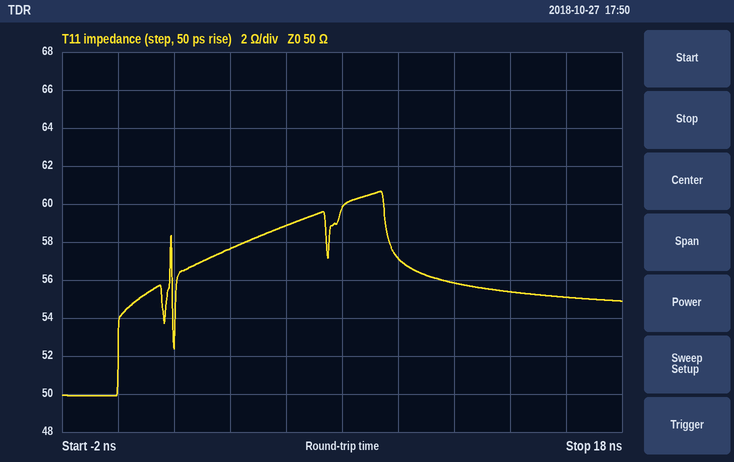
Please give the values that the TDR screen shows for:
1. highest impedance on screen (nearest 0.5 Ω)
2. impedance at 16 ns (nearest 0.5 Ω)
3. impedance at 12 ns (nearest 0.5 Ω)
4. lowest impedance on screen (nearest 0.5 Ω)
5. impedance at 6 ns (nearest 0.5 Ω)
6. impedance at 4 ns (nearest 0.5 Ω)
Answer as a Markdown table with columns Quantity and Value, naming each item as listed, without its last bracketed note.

| Quantity | Value |
|---|---|
| highest impedance on screen | 60.5 Ω |
| impedance at 16 ns | 55.0 Ω |
| impedance at 12 ns | 56.0 Ω |
| lowest impedance on screen | 50.0 Ω |
| impedance at 6 ns | 59.0 Ω |
| impedance at 4 ns | 57.5 Ω |
